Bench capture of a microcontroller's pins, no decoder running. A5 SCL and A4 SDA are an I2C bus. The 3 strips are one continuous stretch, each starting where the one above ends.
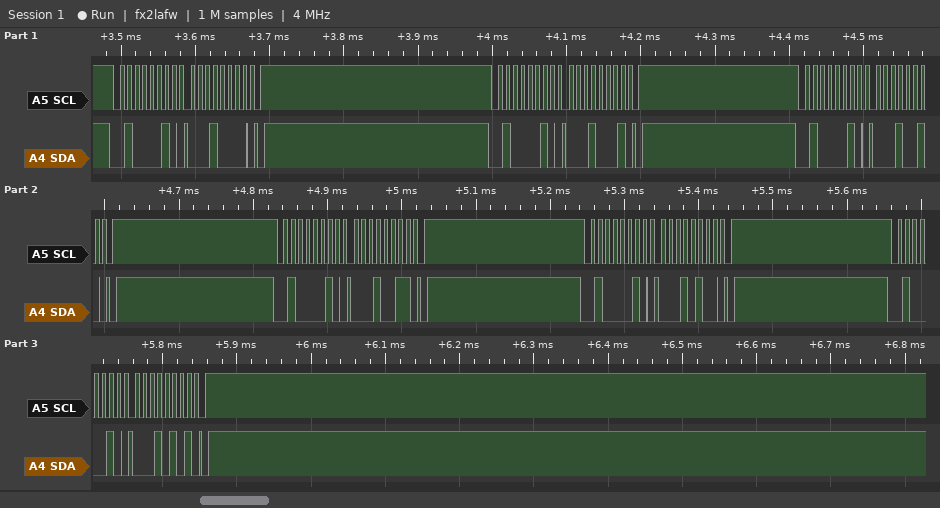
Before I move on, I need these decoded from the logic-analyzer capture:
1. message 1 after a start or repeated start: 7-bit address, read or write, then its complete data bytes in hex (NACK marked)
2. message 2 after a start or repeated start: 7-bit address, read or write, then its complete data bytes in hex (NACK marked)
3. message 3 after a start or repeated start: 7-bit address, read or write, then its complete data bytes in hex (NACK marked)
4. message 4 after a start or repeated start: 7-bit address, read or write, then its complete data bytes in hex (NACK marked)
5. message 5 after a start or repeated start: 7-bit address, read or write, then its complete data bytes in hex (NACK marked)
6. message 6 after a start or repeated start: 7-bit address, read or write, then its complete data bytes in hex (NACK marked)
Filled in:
0x21 write: 10
0x21 write: 11
0x21 write: 12
0x21 write: 13
0x21 write: 14
0x21 write: 15
